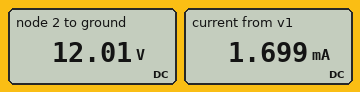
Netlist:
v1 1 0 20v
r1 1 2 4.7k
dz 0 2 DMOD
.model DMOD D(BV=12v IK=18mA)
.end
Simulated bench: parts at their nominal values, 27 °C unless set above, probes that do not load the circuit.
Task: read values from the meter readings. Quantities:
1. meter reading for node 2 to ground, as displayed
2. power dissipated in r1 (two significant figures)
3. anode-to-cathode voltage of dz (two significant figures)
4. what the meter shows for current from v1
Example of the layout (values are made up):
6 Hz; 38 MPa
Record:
12.01 V; 14 mW; -12 V; 1.699 mA
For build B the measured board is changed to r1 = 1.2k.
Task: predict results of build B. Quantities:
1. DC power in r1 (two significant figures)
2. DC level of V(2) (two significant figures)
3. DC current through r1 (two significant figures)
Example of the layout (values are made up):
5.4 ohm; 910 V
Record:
53 mW; 12 V; 6.6 mA
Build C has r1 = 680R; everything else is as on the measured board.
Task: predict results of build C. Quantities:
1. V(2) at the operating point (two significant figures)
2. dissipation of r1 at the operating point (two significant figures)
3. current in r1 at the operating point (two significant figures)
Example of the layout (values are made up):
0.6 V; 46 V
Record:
12 V; 93 mW; 12 mA
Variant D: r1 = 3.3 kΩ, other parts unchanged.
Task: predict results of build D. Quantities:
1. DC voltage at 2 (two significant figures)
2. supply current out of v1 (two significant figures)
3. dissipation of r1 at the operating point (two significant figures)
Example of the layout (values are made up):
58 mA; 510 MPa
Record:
12 V; 2.4 mA; 19 mW
